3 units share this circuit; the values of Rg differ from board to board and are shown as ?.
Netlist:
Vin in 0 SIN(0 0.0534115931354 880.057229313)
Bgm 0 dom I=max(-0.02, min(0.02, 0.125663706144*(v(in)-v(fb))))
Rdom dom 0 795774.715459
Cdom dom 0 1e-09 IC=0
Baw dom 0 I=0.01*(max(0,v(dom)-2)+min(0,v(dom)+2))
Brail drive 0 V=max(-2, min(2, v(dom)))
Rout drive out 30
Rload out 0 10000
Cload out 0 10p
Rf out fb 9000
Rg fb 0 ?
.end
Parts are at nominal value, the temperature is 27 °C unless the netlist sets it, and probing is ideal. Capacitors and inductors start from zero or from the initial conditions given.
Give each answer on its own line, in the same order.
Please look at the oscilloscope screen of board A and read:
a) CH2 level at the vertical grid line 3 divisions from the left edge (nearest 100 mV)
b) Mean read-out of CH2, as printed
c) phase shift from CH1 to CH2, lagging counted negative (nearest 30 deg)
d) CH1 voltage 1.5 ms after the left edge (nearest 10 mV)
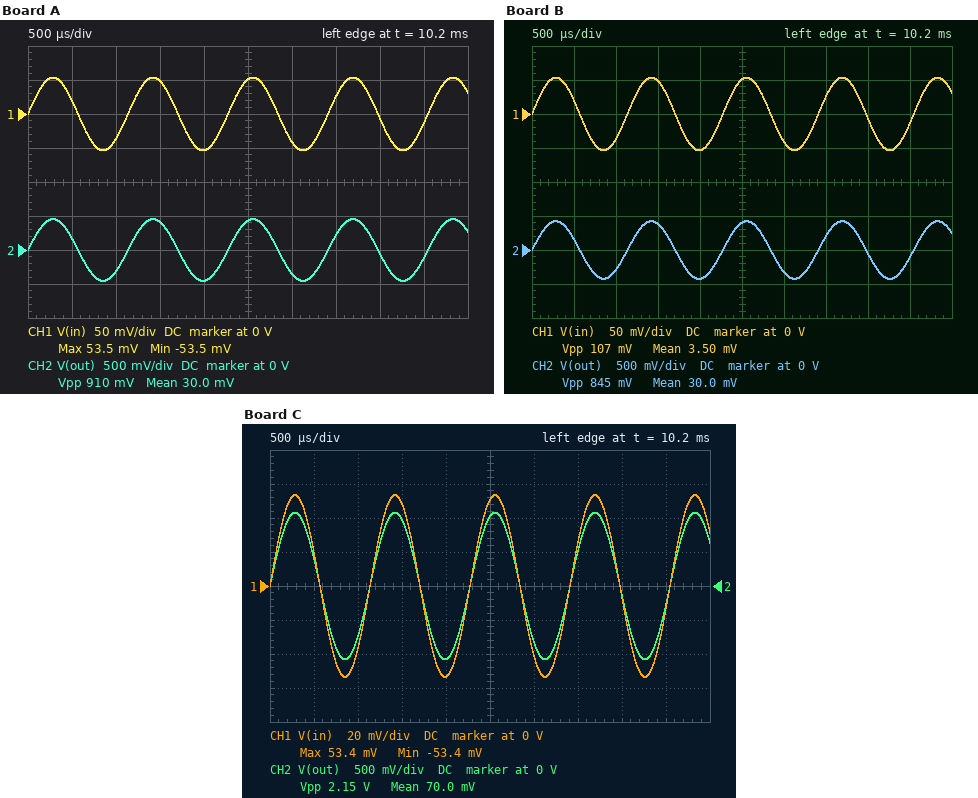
400 mV
30.0 mV
0 deg
50 mV
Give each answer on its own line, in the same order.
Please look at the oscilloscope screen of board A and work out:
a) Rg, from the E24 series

1.2 kΩ
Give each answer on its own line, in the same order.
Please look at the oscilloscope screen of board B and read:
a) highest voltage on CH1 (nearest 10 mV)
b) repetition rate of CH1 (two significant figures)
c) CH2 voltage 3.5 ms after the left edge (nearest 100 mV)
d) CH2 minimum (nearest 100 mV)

50 mV
880 Hz
200 mV
-400 mV
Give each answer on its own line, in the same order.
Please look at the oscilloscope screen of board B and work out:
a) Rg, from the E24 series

1.3 kΩ
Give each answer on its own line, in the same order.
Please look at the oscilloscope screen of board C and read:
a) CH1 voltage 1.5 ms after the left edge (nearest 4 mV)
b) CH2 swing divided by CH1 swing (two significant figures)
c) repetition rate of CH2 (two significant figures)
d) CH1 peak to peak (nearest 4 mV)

48 mV
20
880 Hz
108 mV
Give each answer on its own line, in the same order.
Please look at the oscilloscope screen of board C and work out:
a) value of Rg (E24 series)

470 Ω
